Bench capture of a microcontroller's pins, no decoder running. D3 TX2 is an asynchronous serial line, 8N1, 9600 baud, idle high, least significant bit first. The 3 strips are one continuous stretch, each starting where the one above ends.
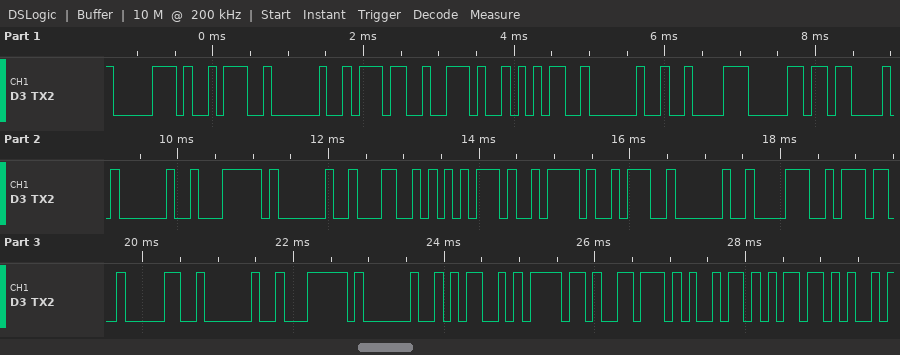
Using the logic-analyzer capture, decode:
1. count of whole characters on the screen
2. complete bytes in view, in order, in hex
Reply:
29
70 3A 20 37 2E 35 20 C2 B0 43 20 7C 20 4C 75 7A 3A 20 38 37 30 20 7C 20 4D 6F 76 69 6D
